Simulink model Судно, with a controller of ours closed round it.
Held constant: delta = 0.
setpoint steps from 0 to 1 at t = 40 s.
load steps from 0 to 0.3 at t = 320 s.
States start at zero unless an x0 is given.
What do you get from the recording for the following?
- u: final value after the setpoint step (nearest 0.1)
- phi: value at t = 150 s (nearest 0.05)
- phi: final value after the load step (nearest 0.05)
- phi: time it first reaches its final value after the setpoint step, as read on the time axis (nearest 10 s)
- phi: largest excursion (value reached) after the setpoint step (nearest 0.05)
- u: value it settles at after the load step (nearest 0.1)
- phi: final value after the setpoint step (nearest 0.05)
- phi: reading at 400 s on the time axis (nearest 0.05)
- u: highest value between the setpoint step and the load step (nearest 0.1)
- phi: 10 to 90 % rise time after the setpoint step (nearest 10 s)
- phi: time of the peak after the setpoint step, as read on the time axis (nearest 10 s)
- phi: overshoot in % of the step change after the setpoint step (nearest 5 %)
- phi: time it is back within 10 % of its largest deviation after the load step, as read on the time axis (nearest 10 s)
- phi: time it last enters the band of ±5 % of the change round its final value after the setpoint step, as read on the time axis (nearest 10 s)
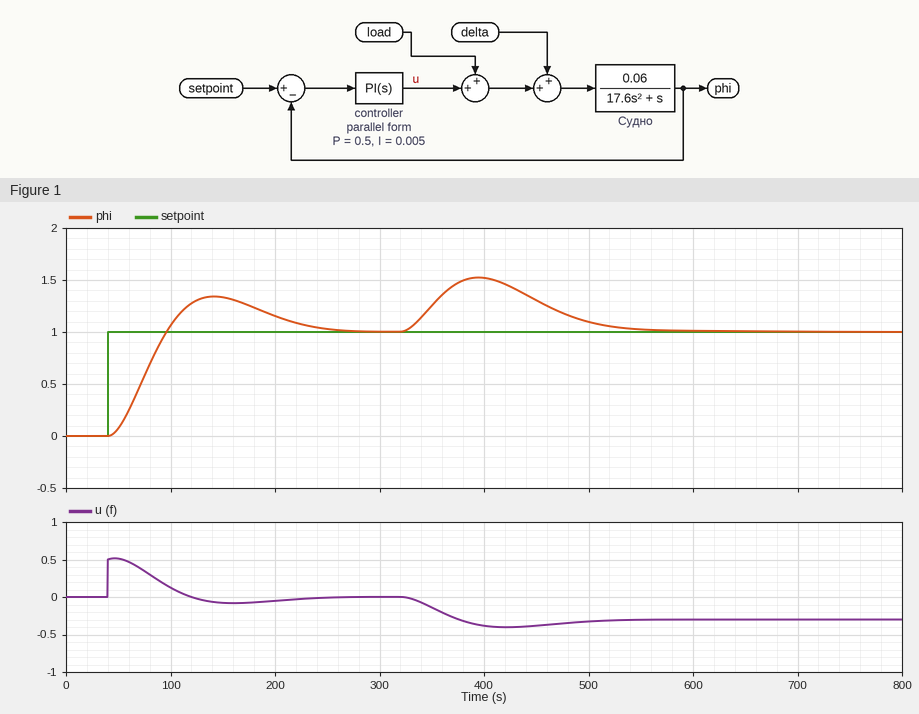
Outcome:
0.0
1.35
1.00
100 s
1.35
-0.3
1.00
1.50
0.5
40 s
140 s
35 %
520 s
240 s
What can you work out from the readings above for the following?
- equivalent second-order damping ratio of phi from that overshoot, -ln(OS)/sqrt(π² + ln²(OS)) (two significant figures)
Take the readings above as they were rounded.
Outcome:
0.32
